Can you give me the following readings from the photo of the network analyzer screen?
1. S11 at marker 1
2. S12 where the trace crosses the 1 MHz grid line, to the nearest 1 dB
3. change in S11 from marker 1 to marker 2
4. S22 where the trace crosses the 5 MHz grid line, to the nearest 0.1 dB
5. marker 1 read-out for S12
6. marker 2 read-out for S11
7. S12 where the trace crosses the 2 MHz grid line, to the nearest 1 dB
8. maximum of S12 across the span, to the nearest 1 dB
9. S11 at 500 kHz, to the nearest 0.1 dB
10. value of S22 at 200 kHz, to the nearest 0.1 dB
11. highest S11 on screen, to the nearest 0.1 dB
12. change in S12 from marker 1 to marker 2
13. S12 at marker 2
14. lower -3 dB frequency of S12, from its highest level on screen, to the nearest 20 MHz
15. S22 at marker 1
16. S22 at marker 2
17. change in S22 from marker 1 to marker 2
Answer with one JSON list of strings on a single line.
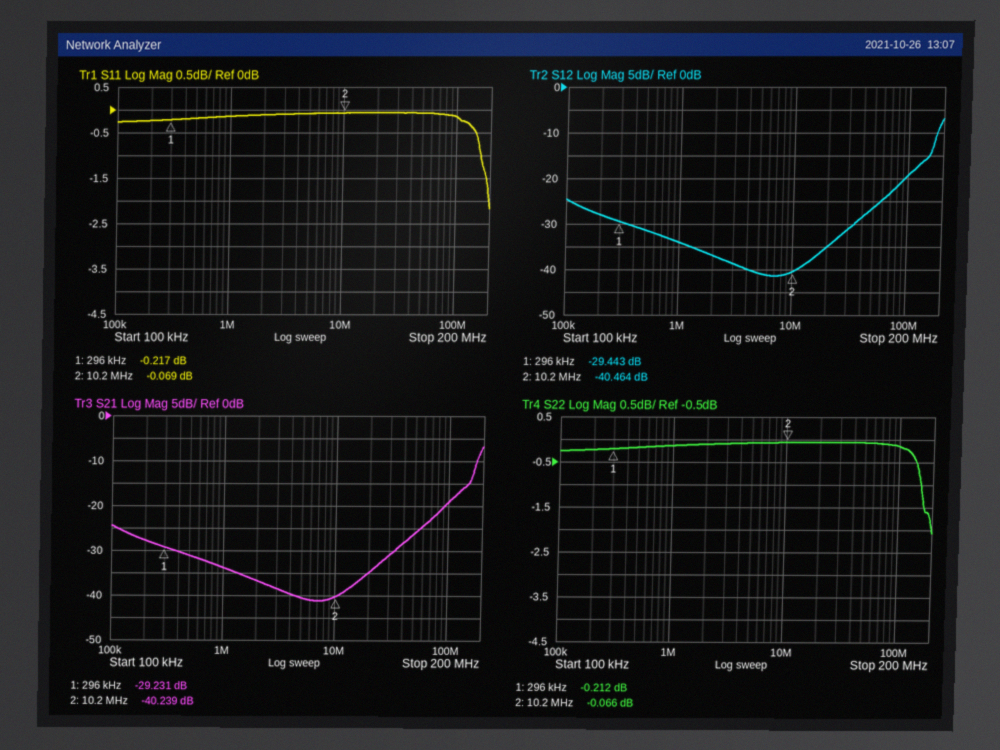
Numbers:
["-0.217 dB", "-34 dB", "0.148 dB", "-0.1 dB", "-29.443 dB", "-0.069 dB", "-37 dB", "-7 dB", "-0.2 dB", "-0.2 dB", "-0.1 dB", "-11.021 dB", "-40.464 dB", "180 MHz", "-0.212 dB", "-0.066 dB", "0.146 dB"]
